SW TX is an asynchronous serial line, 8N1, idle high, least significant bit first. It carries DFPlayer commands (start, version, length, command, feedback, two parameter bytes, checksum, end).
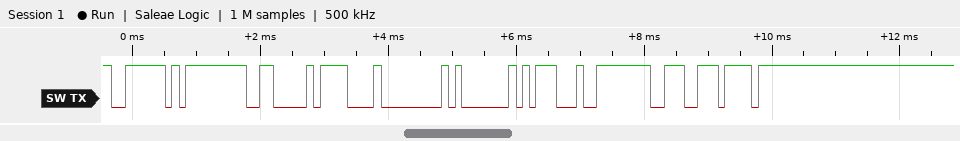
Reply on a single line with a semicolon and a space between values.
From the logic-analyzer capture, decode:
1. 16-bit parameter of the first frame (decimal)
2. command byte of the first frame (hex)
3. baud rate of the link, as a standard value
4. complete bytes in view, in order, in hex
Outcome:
285; 0x0F; 9600 baud; 0x7E 0xFF 0x06 0x0F 0x00 0x01 0x1D 0xFE 0xCE 0xEF
